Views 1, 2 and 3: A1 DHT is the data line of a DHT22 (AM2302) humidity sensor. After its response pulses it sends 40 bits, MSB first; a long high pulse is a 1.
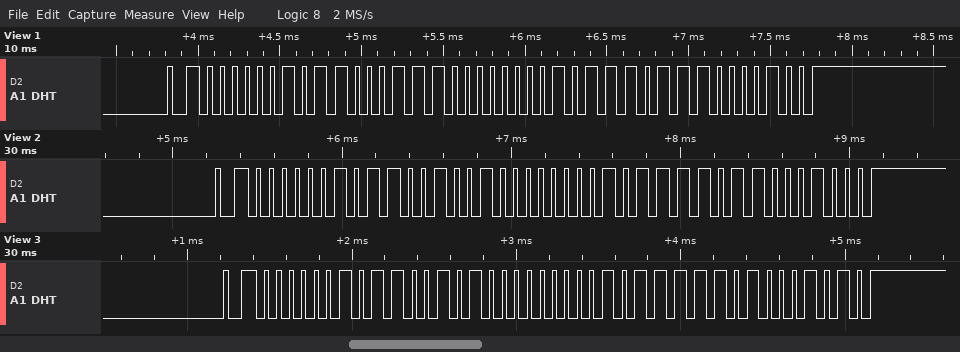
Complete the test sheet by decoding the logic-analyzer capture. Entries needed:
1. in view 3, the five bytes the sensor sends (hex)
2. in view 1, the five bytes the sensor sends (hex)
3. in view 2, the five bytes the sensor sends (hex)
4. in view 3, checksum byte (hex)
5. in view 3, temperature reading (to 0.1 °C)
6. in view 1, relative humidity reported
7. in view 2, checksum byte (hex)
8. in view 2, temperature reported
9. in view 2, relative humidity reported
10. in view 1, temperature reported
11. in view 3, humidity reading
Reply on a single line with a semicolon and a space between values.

02 CA 00 BE 8A; 02 C7 00 BB 84; 02 C9 00 BD 88; 0x8A; 19.0 °C; 71.1 %; 0x88; 18.9 °C; 71.3 %; 18.7 °C; 71.4 %
